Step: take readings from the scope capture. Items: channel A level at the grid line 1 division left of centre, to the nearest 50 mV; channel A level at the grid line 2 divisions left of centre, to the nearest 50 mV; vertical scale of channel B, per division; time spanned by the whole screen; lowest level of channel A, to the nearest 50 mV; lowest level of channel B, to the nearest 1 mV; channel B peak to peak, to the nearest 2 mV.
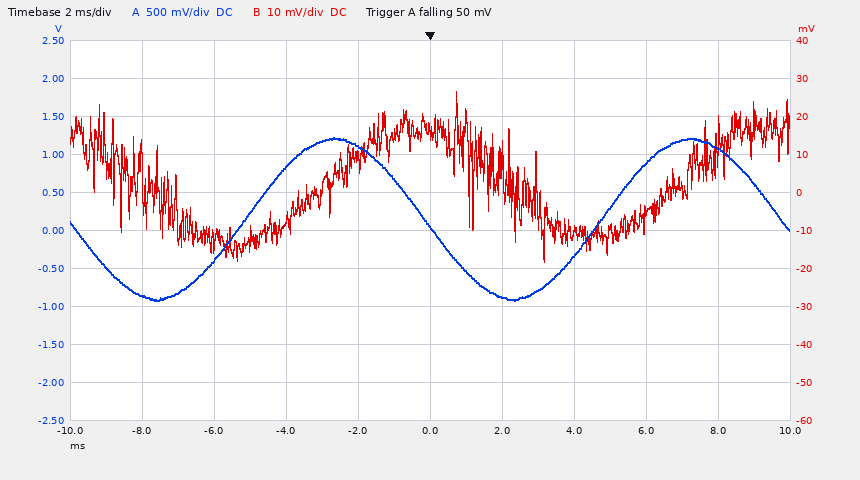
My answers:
1.10 V
850 mV
10 mV
20 ms
-900 mV
-18 mV
44 mV
